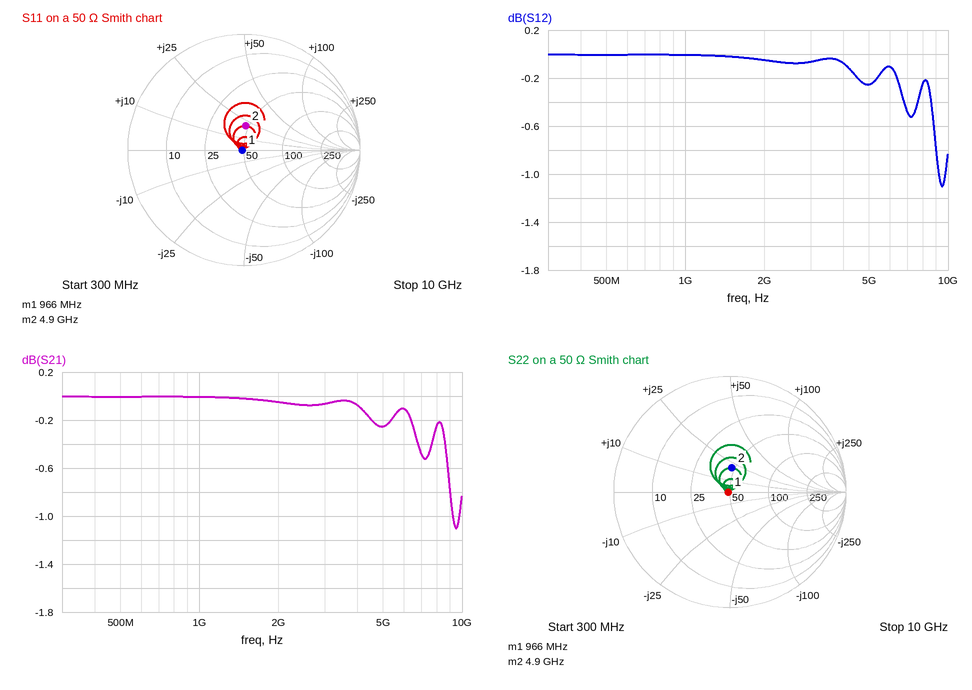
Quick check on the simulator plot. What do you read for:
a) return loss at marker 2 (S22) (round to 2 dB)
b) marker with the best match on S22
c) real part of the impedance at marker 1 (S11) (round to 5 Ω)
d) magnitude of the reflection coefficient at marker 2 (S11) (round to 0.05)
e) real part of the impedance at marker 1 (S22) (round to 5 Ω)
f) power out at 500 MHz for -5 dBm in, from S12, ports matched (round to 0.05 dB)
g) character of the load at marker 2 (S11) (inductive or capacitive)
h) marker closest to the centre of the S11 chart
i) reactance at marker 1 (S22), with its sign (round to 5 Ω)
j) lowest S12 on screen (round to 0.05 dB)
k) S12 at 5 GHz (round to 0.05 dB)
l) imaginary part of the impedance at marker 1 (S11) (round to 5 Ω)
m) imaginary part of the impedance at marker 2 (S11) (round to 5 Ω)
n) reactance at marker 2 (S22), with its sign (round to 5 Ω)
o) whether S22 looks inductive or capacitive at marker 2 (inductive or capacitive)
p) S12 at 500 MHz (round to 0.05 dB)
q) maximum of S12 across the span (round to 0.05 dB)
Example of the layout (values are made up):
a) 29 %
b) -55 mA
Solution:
a) 14 dB
b) marker 1
c) 50 Ω
d) 0.20
e) 50 Ω
f) -5.00 dBm
g) inductive
h) marker 1
i) 0 Ω
j) -1.10 dB
k) -0.25 dB
l) 0 Ω
m) +20 Ω
n) +20 Ω
o) inductive
p) 0.00 dB
q) 0.00 dB
